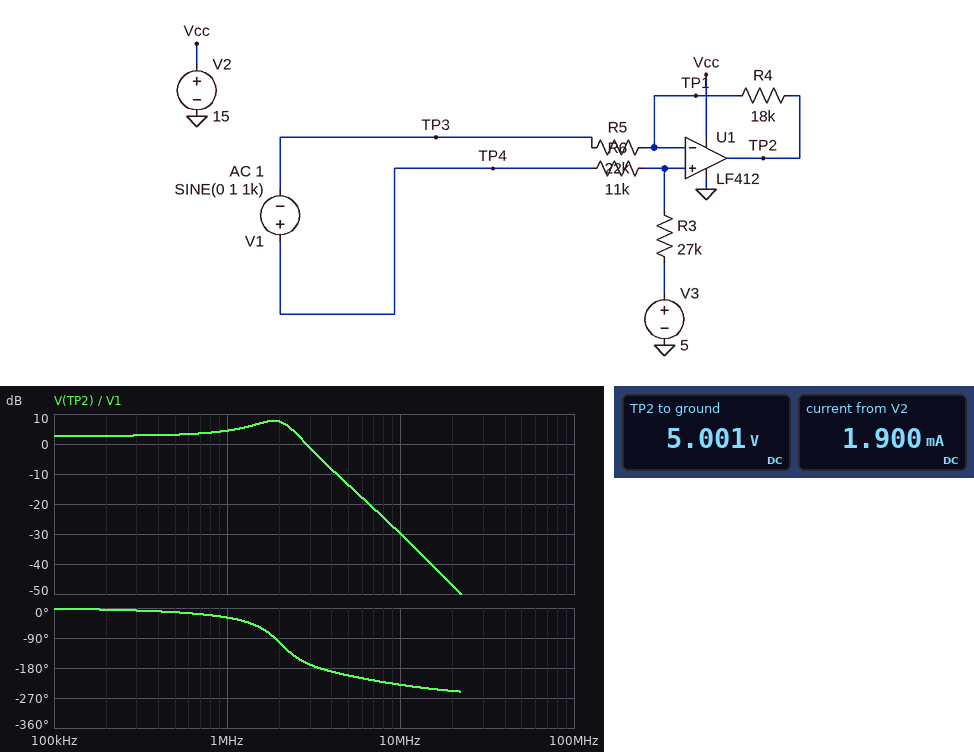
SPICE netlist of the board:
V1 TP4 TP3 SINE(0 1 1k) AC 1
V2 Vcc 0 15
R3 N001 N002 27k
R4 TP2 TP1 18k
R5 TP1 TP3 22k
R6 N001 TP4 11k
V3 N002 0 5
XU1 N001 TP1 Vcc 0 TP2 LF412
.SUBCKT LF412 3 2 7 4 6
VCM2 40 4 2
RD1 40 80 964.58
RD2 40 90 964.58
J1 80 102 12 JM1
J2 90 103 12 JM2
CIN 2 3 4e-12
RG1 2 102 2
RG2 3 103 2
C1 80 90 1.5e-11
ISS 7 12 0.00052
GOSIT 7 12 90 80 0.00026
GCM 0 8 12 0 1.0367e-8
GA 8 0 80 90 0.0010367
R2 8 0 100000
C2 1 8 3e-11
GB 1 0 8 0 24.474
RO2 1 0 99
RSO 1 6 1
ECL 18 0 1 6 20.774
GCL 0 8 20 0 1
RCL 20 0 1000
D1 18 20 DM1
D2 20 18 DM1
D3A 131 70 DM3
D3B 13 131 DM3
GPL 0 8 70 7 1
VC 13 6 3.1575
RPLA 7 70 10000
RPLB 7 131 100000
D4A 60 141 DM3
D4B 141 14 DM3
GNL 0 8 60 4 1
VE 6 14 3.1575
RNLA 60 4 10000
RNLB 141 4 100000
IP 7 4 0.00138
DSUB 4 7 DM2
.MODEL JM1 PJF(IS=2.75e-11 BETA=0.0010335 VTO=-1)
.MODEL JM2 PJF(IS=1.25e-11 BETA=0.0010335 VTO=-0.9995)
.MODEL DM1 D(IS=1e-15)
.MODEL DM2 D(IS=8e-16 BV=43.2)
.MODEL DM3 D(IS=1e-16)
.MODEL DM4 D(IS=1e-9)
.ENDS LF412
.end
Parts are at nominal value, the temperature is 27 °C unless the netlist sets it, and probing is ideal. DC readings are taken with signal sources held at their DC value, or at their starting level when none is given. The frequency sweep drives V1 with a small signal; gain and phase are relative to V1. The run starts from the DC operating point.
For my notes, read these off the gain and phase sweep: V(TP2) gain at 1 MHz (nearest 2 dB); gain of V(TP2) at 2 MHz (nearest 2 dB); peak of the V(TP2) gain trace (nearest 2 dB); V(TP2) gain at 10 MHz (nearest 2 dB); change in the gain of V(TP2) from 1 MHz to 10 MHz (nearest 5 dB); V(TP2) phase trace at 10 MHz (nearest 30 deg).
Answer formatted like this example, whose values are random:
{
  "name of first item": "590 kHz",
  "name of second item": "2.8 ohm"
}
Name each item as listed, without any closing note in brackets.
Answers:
{
  "V(TP2) gain at 1 MHz": "4 dB",
  "gain of V(TP2) at 2 MHz": "8 dB",
  "peak of the V(TP2) gain trace": "8 dB",
  "V(TP2) gain at 10 MHz": "-30 dB",
  "change in the gain of V(TP2) from 1 MHz to 10 MHz": "-35 dB",
  "V(TP2) phase trace at 10 MHz": "-240 deg"
}
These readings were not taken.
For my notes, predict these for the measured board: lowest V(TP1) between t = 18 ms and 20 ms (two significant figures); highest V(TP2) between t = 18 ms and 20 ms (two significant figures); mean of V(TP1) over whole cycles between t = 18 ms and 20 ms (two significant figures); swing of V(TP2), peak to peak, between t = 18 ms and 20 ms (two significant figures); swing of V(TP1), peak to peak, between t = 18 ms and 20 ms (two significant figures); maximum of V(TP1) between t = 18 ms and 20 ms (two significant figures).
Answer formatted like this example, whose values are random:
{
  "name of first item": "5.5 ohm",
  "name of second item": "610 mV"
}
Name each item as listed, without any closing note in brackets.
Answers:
{
  "lowest V(TP1) between t = 18 ms and 20 ms": "4.2 V",
  "highest V(TP2) between t = 18 ms and 20 ms": "6.4 V",
  "mean of V(TP1) over whole cycles between t = 18 ms and 20 ms": "5.0 V",
  "swing of V(TP2), peak to peak, between t = 18 ms and 20 ms": "2.7 V",
  "swing of V(TP1), peak to peak, between t = 18 ms and 20 ms": "1.6 V",
  "maximum of V(TP1) between t = 18 ms and 20 ms": "5.8 V"
}
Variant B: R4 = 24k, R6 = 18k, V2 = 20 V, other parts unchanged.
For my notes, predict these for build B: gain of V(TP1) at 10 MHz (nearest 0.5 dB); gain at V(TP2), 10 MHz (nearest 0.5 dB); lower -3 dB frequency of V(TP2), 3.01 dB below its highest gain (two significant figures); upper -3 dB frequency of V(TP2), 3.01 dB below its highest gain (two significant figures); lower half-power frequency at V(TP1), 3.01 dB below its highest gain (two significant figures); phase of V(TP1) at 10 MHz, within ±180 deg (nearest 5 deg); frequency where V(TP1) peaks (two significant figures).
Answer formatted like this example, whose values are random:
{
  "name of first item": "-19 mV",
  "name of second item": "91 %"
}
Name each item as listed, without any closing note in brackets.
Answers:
{
  "gain of V(TP1) at 10 MHz": "-24.5 dB",
  "gain at V(TP2), 10 MHz": "-31.5 dB",
  "lower -3 dB frequency of V(TP2), 3.01 dB below its highest gain": "1.2 MHz",
  "upper -3 dB frequency of V(TP2), 3.01 dB below its highest gain": "2.2 MHz",
  "lower half-power frequency at V(TP1), 3.01 dB below its highest gain": "1.3 MHz",
  "phase of V(TP1) at 10 MHz, within ±180 deg": "105 deg",
  "frequency where V(TP1) peaks": "1.8 MHz"
}
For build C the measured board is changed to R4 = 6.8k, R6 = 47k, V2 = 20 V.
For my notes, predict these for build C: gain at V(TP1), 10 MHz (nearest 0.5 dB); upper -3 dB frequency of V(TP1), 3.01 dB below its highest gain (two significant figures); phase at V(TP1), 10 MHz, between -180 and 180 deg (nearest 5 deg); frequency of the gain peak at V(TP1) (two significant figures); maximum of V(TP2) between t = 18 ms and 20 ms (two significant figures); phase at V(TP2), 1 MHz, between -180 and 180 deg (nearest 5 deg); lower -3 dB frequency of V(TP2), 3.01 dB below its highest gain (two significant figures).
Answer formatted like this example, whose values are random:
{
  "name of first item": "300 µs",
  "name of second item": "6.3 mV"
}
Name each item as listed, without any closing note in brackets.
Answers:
{
  "gain at V(TP1), 10 MHz": "-32.5 dB",
  "upper -3 dB frequency of V(TP1), 3.01 dB below its highest gain": "2.6 MHz",
  "phase at V(TP1), 10 MHz, between -180 and 180 deg": "115 deg",
  "frequency of the gain peak at V(TP1)": "2.3 MHz",
  "maximum of V(TP2) between t = 18 ms and 20 ms": "5.5 V",
  "phase at V(TP2), 1 MHz, between -180 and 180 deg": "-15 deg",
  "lower -3 dB frequency of V(TP2), 3.01 dB below its highest gain": "1.9 MHz"
}
